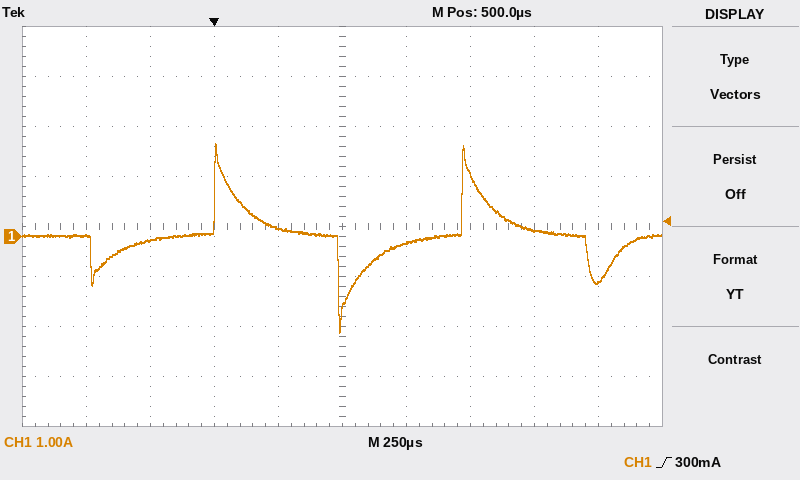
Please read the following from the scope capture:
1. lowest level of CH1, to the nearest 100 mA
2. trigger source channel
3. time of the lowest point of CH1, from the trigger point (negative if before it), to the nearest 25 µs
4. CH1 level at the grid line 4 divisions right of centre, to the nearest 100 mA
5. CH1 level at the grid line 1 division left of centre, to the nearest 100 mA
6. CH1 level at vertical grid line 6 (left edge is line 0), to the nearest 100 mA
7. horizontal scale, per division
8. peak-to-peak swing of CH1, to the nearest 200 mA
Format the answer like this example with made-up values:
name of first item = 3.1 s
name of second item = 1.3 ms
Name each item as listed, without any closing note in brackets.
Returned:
lowest level of CH1, to the nearest 100 mA = -1.9 A
trigger source channel = CH1
time of the lowest point of CH1, from the trigger point (negative if before it), to the nearest 25 µs = +500 µs
CH1 level at the grid line 4 divisions right of centre, to the nearest 100 mA = -900 mA
CH1 level at the grid line 1 division left of centre, to the nearest 100 mA = 200 mA
CH1 level at vertical grid line 6 (left edge is line 0), to the nearest 100 mA = -100 mA
horizontal scale, per division = 250 µs
peak-to-peak swing of CH1, to the nearest 200 mA = 3.8 A
